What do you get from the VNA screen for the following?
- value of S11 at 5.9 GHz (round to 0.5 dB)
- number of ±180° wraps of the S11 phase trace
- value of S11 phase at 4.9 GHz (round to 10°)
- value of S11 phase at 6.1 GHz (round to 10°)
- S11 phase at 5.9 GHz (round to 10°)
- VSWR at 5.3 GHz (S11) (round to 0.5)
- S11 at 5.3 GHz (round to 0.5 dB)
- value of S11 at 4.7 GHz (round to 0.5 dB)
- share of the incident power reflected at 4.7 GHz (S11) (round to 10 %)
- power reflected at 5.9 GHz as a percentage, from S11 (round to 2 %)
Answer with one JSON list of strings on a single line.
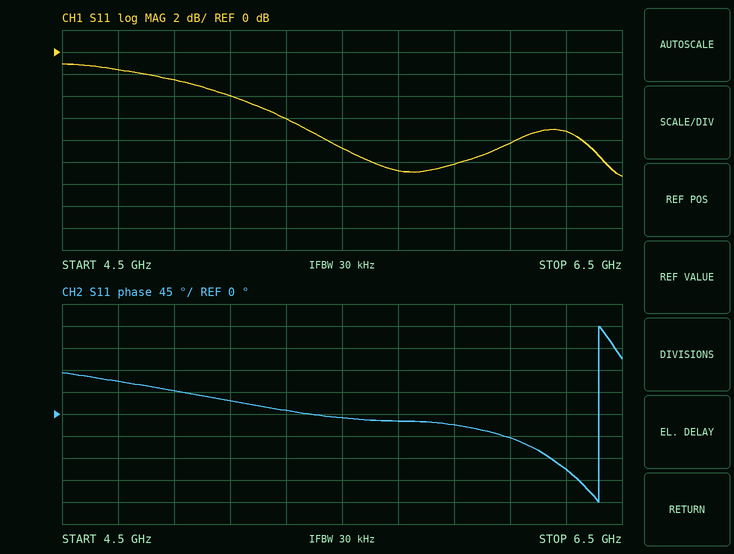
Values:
["-10.0 dB", "1", "50°", "-50°", "-20°", "3.0", "-6.0 dB", "-1.5 dB", "70 %", "10 %"]
